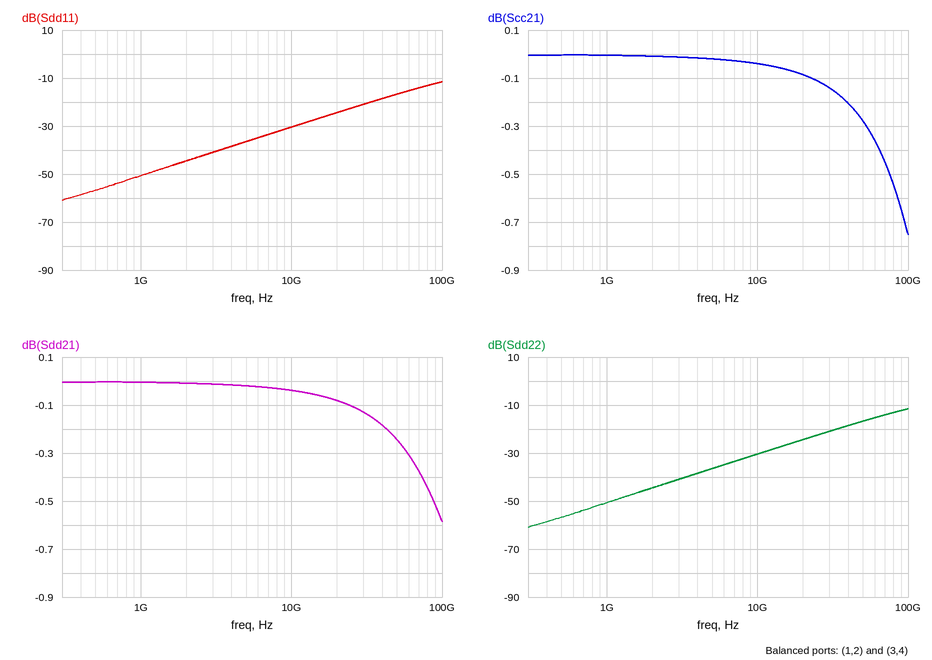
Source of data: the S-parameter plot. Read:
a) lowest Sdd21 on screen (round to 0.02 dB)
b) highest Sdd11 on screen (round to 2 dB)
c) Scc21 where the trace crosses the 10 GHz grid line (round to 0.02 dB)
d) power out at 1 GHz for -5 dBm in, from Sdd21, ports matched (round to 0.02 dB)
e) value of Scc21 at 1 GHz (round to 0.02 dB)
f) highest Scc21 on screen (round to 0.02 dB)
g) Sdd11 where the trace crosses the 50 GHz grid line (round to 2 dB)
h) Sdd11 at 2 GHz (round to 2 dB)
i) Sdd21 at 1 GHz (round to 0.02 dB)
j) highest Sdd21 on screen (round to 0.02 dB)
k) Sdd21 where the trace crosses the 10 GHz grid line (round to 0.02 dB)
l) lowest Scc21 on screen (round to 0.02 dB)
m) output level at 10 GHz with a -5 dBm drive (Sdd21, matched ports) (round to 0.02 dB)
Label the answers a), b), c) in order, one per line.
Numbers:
a) -0.58 dB
b) -12 dB
c) -0.04 dB
d) -5.00 dBm
e) 0.00 dB
f) 0.00 dB
g) -16 dB
h) -44 dB
i) 0.00 dB
j) 0.00 dB
k) -0.04 dB
l) -0.76 dB
m) -5.04 dBm
